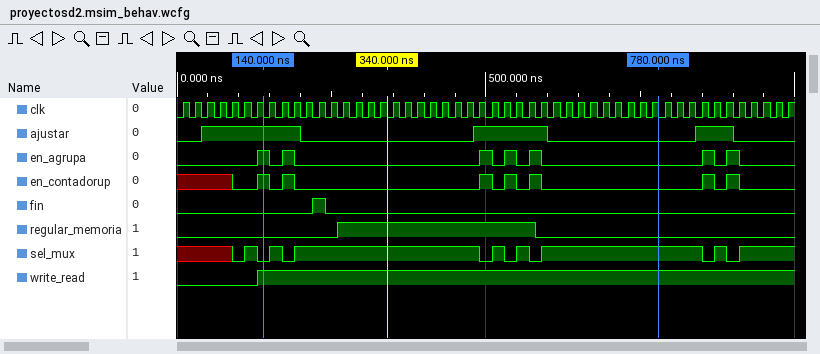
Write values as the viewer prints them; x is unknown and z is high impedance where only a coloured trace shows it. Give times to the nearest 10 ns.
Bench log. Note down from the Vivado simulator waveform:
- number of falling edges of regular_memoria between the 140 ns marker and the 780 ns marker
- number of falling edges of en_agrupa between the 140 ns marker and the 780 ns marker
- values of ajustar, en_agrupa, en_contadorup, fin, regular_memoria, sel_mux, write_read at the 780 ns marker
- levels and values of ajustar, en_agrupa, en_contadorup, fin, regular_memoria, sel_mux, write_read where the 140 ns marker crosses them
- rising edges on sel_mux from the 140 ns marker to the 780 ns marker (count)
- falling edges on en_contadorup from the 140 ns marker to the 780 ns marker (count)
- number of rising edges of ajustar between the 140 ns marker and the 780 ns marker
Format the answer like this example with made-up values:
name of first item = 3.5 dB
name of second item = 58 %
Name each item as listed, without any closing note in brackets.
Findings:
number of falling edges of regular_memoria between the 140 ns marker and the 780 ns marker = 1
number of falling edges of en_agrupa between the 140 ns marker and the 780 ns marker = 5
values of ajustar, en_agrupa, en_contadorup, fin, regular_memoria, sel_mux, write_read at the 780 ns marker = ajustar=0, en_agrupa=0, en_contadorup=0, fin=0, regular_memoria=0, sel_mux=1, write_read=1
levels and values of ajustar, en_agrupa, en_contadorup, fin, regular_memoria, sel_mux, write_read where the 140 ns marker crosses them = ajustar=1, en_agrupa=1, en_contadorup=1, fin=0, regular_memoria=0, sel_mux=0, write_read=1
rising edges on sel_mux from the 140 ns marker to the 780 ns marker = 5
falling edges on en_contadorup from the 140 ns marker to the 780 ns marker = 5
number of rising edges of ajustar between the 140 ns marker and the 780 ns marker = 1
